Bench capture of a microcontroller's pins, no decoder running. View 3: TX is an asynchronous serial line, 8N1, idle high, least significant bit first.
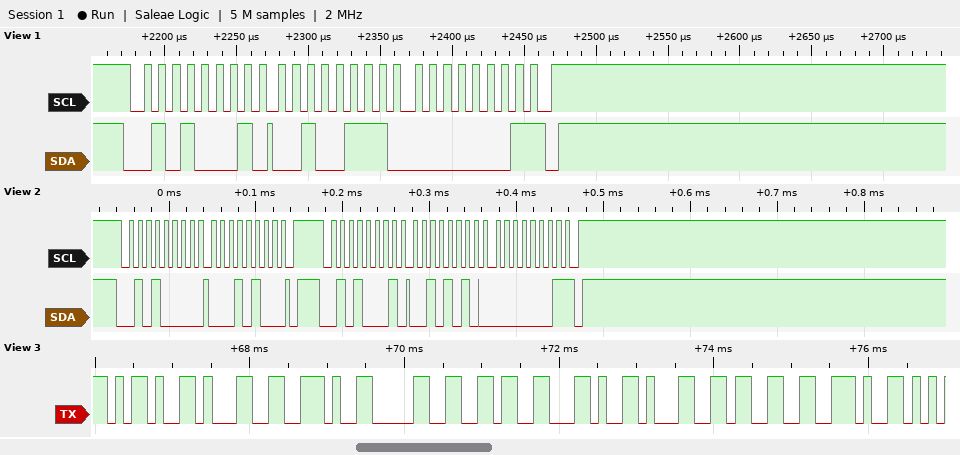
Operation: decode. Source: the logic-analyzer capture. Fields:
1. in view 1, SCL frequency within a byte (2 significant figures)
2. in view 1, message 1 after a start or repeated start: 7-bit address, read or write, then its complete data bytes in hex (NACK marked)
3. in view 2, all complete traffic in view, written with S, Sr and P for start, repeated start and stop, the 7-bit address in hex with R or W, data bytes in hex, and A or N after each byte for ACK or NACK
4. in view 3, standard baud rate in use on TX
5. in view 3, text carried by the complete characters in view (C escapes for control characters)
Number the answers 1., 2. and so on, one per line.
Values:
1. 100 kHz
2. 0x28 read: 27 01 NACK
3. S 28W A 14 A P S 28R A 2A A 01 N P
4. 9600 baud
5. "-1.06,13."
